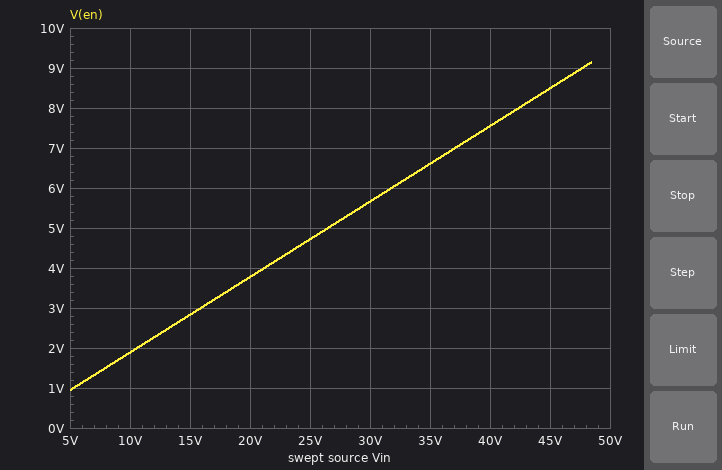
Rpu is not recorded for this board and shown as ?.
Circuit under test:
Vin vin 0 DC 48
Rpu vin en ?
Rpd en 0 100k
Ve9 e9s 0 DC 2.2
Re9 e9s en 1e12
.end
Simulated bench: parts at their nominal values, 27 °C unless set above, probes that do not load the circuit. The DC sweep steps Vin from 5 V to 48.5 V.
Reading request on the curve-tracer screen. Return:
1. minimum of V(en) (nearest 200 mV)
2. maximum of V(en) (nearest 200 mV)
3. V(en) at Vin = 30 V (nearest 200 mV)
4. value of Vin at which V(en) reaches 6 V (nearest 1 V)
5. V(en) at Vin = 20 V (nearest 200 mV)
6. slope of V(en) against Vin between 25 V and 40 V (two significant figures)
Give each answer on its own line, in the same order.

1.0 V
9.2 V
5.6 V
32 V
3.8 V
0.19 V/V
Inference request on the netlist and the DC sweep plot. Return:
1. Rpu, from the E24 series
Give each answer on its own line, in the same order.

430 kΩ
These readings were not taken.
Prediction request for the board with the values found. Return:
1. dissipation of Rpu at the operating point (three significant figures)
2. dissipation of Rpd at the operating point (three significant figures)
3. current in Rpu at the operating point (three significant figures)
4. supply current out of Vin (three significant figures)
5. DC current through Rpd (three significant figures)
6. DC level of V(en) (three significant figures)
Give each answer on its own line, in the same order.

3.53 mW
820 µW
90.6 µA
90.6 µA
90.6 µA
9.06 V
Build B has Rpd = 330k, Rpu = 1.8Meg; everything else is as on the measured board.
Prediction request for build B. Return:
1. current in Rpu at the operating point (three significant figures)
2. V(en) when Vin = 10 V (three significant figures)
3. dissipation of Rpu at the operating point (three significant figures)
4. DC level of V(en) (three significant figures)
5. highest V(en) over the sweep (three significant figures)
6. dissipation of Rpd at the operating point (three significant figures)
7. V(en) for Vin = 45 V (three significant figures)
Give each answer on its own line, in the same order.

22.5 µA
1.55 V
914 µW
7.44 V
7.51 V
168 µW
6.97 V
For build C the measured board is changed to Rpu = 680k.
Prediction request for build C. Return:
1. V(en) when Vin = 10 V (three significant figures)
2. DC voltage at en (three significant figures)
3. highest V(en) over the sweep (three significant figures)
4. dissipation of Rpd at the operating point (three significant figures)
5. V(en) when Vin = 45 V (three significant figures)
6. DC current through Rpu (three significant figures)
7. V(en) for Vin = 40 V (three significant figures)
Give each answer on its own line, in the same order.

1.28 V
6.15 V
6.22 V
379 µW
5.77 V
61.5 µA
5.13 V
